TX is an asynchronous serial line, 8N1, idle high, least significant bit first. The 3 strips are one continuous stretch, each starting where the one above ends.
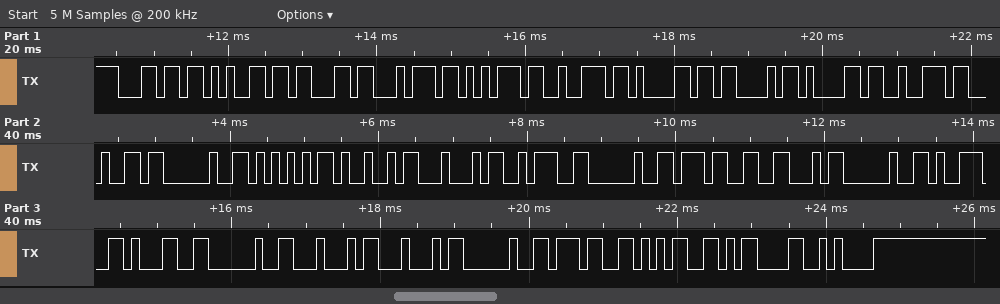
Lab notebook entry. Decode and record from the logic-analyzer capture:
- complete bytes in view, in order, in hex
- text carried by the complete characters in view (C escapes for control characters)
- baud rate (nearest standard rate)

6C 65 63 74 75 72 61 43 61 72 64 20 55 49 44 3A 20 37 46 20 39 31 20 44 44 20 37 35 0D 0A
"lecturaCard UID: 7F 91 DD 75\r\n"
9600 baud
